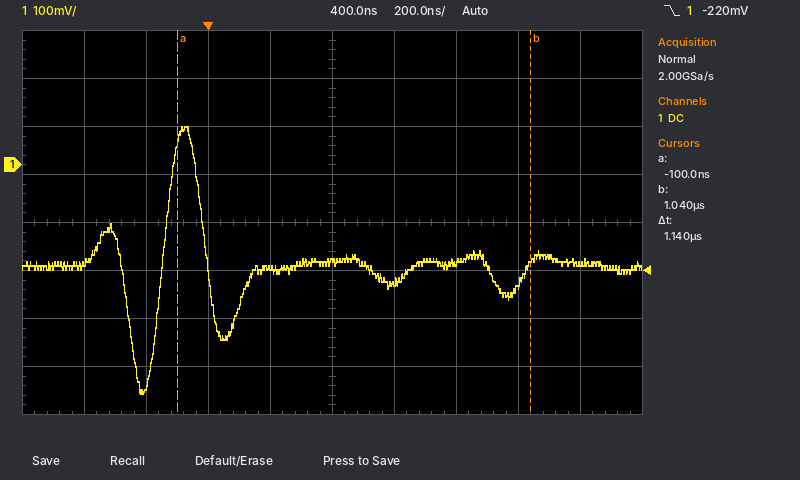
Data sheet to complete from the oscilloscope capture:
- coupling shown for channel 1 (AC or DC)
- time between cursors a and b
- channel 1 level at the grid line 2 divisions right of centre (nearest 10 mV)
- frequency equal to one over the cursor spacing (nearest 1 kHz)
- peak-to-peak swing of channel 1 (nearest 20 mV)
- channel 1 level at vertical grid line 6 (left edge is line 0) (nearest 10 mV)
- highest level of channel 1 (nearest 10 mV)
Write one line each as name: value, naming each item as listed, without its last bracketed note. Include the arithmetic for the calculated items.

coupling shown for channel 1: DC
time between cursors a and b: 1.14 µs
channel 1 level at the grid line 2 divisions right of centre: -200 mV
frequency equal to one over the cursor spacing: 1 / 1.14 µs ≈ 877 kHz
peak-to-peak swing of channel 1: 560 mV
channel 1 level at vertical grid line 6 (left edge is line 0): -240 mV
highest level of channel 1: 80 mV
